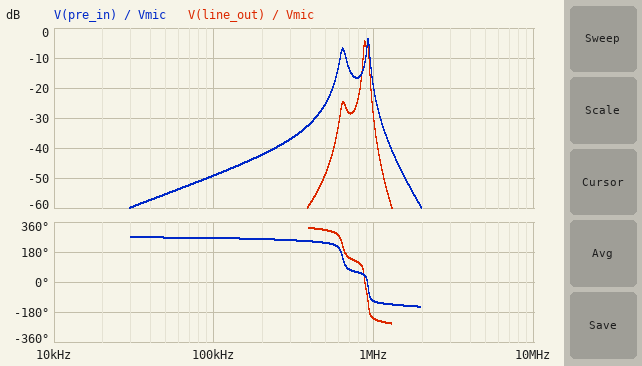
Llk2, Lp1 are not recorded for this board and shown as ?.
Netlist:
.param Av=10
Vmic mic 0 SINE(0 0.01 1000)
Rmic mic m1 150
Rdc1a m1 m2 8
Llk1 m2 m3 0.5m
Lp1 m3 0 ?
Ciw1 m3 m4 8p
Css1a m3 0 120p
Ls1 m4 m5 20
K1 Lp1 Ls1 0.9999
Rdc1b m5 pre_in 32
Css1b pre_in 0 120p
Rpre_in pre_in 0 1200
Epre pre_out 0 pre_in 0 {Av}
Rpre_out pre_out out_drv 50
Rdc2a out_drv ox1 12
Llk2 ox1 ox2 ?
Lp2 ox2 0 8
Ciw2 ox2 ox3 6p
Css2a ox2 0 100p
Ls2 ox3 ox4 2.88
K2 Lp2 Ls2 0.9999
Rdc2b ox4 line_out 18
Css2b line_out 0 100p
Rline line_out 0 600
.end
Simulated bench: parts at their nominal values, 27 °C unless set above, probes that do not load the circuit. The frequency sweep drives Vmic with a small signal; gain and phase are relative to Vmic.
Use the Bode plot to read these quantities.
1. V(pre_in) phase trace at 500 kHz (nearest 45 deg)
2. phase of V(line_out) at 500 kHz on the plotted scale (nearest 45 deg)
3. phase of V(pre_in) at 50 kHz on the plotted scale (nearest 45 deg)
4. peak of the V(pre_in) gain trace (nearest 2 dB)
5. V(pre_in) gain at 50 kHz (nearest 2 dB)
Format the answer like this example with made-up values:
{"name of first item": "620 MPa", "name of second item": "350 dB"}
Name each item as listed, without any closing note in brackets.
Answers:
{"V(pre_in) phase trace at 500 kHz": "225 deg", "phase of V(line_out) at 500 kHz on the plotted scale": "315 deg", "phase of V(pre_in) at 50 kHz on the plotted scale": "270 deg", "peak of the V(pre_in) gain trace": "-4 dB", "V(pre_in) gain at 50 kHz": "-56 dB"}
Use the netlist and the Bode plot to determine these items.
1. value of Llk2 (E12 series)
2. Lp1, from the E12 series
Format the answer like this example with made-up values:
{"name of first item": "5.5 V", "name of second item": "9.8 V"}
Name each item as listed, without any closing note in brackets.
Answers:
{"value of Llk2": "330 µH", "Lp1, from the E12 series": "8.2 H"}
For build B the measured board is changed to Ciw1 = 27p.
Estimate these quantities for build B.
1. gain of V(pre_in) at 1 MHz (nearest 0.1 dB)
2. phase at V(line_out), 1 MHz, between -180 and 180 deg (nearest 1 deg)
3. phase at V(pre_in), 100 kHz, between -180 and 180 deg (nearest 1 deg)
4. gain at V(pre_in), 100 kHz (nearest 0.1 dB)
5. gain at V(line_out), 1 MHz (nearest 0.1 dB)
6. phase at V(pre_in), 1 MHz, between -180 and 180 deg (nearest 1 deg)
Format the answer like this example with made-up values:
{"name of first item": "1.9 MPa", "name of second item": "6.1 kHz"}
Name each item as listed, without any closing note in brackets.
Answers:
{"gain of V(pre_in) at 1 MHz": "-33.9 dB", "phase at V(line_out), 1 MHz, between -180 and 180 deg": "130 deg", "phase at V(pre_in), 100 kHz, between -180 and 180 deg": "-97 deg", "gain at V(pre_in), 100 kHz": "-38.3 dB", "gain at V(line_out), 1 MHz": "-44.2 dB", "phase at V(pre_in), 1 MHz, between -180 and 180 deg": "-125 deg"}
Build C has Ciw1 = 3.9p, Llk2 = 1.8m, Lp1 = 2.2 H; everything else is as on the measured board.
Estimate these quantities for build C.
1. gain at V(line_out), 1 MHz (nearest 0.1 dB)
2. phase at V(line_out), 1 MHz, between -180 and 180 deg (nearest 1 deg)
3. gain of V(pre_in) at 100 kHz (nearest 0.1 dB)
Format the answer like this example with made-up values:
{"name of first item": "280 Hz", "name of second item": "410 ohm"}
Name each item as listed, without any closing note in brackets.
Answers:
{"gain at V(line_out), 1 MHz": "-61.9 dB", "phase at V(line_out), 1 MHz, between -180 and 180 deg": "-61 deg", "gain of V(pre_in) at 100 kHz": "-44.3 dB"}
